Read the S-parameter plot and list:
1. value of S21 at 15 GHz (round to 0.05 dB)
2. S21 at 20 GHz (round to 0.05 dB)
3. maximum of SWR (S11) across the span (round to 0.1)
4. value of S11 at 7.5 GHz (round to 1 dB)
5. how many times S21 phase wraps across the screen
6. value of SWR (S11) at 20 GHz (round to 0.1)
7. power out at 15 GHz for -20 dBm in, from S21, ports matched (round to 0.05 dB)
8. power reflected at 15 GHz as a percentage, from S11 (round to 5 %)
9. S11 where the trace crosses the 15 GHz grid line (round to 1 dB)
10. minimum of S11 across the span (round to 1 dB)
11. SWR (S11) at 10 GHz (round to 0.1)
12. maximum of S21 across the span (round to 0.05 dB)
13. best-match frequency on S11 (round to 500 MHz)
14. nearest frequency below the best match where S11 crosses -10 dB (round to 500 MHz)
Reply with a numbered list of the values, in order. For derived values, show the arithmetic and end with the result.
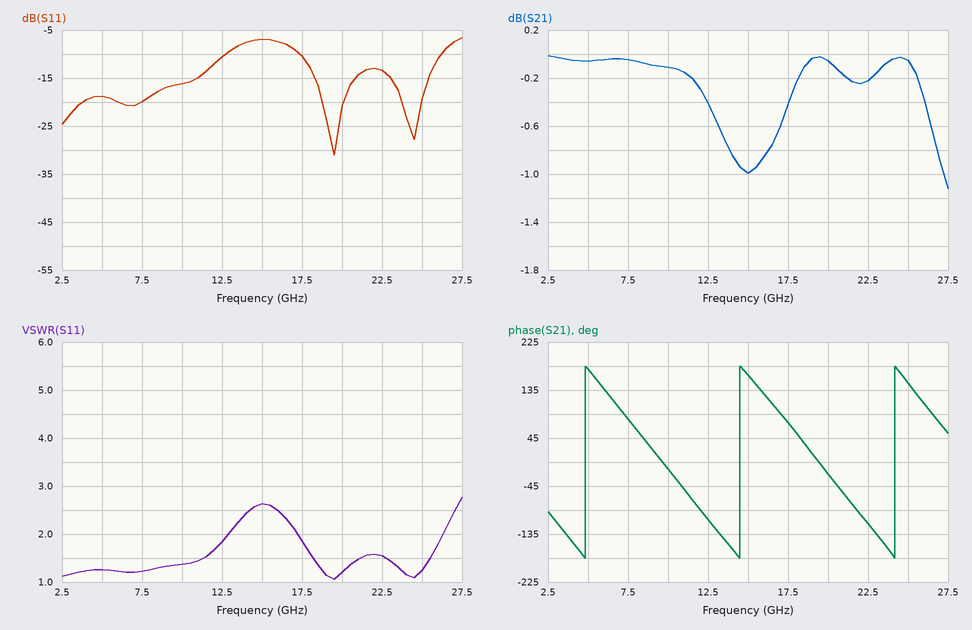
1. -1.00 dB
2. -0.05 dB
3. 2.8
4. -20 dB
5. 3
6. 1.2
7. -20 dBm + (-1.00 dB) = -21.00 dBm
8. 10^(-7/10) ≈ 20 %
9. -7 dB
10. -31 dB
11. 1.4
12. 0.00 dB
13. 19.5 GHz
14. 17.5 GHz
